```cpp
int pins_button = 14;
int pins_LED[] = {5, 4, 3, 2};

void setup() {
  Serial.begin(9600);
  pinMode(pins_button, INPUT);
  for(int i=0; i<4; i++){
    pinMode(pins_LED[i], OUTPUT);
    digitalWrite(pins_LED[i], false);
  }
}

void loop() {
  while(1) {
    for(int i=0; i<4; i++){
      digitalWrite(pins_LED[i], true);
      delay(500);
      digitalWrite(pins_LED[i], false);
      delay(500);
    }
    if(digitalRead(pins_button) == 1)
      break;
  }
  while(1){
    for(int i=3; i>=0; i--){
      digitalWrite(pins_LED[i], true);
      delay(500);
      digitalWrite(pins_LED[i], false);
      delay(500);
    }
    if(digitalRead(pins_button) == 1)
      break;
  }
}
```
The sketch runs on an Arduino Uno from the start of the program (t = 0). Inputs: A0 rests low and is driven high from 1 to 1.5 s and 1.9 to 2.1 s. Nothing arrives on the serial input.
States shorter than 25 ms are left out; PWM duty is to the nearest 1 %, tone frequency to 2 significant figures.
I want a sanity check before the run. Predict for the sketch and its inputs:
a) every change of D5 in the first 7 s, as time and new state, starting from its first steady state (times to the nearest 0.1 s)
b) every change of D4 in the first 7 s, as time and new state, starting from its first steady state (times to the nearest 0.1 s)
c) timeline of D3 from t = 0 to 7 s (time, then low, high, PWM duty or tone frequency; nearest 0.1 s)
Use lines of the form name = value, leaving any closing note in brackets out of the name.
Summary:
every change of D5 in the first 7 s, as time and new state, starting from its first steady state = 0 s high; 0.5 s low; 4 s high; 4.5 s low
every change of D4 in the first 7 s, as time and new state, starting from its first steady state = 0 s low; 1 s high; 1.5 s low; 5 s high; 5.5 s low
timeline of D3 from t = 0 to 7 s = 0 s low; 2 s high; 2.5 s low; 6 s high; 6.5 s low
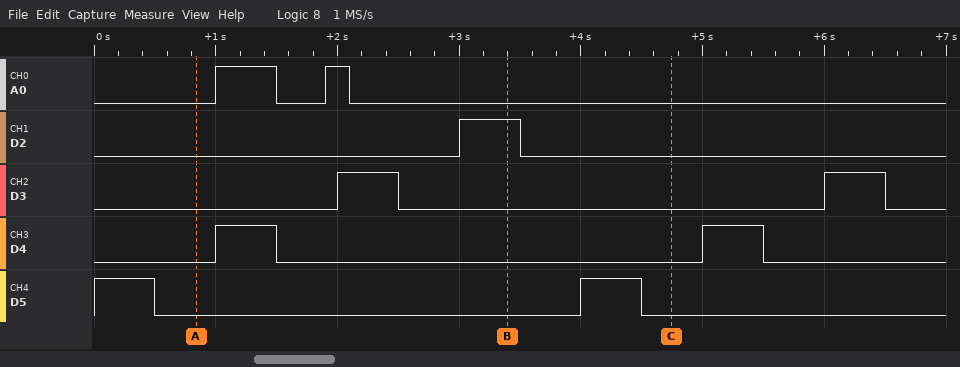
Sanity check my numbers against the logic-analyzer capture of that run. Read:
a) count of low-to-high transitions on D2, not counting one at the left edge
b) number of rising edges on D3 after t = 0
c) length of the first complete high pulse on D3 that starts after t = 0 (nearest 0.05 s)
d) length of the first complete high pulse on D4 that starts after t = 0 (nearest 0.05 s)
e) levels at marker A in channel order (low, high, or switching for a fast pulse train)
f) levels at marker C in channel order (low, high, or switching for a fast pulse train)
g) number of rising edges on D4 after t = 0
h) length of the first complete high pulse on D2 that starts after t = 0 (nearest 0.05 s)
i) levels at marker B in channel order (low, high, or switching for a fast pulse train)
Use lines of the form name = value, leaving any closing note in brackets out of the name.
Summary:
count of low-to-high transitions on D2, not counting one at the left edge = 1
number of rising edges on D3 after t = 0 = 2
length of the first complete high pulse on D3 that starts after t = 0 = 0.50 s
length of the first complete high pulse on D4 that starts after t = 0 = 0.50 s
levels at marker A in channel order = A0 low, D2 low, D3 low, D4 low, D5 low
levels at marker C in channel order = A0 low, D2 low, D3 low, D4 low, D5 low
number of rising edges on D4 after t = 0 = 2
length of the first complete high pulse on D2 that starts after t = 0 = 0.50 s
levels at marker B in channel order = A0 low, D2 high, D3 low, D4 low, D5 low
